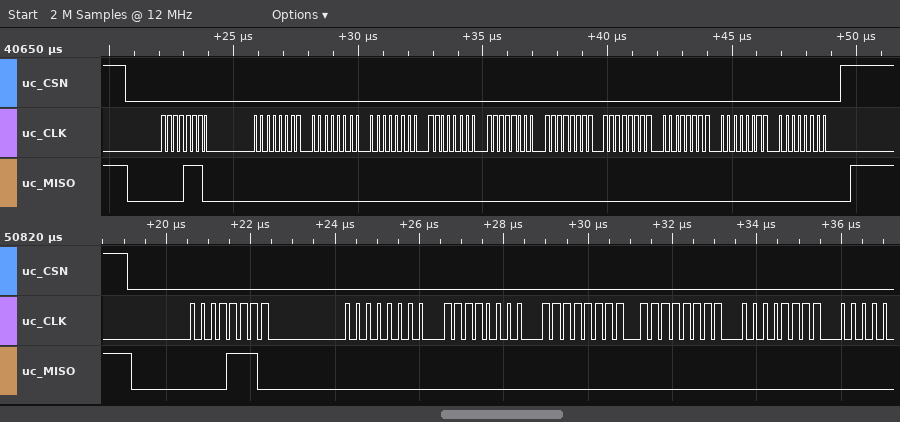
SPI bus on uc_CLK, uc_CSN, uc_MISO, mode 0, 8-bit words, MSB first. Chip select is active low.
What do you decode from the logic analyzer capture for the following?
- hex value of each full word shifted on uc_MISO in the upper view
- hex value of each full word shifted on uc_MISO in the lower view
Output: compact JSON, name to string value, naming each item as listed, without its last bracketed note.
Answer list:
{"hex value of each full word shifted on uc_MISO in the upper view": "0E, 00, 00, 00, 00, 00, 00, 00, 00, 00, 00", "hex value of each full word shifted on uc_MISO in the lower view": "0E, 00, 00, 00, 00, 00"}
